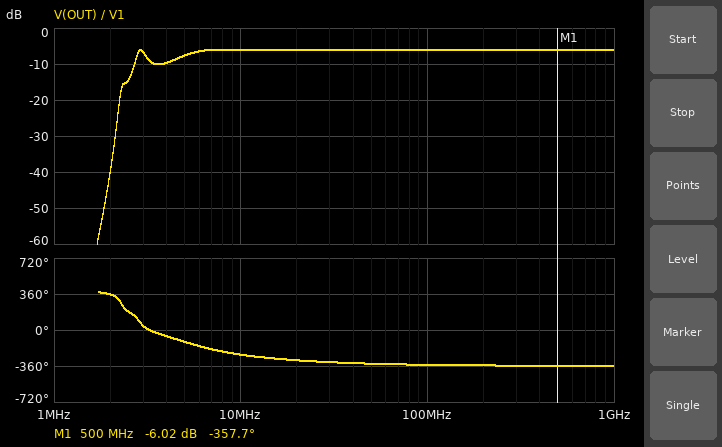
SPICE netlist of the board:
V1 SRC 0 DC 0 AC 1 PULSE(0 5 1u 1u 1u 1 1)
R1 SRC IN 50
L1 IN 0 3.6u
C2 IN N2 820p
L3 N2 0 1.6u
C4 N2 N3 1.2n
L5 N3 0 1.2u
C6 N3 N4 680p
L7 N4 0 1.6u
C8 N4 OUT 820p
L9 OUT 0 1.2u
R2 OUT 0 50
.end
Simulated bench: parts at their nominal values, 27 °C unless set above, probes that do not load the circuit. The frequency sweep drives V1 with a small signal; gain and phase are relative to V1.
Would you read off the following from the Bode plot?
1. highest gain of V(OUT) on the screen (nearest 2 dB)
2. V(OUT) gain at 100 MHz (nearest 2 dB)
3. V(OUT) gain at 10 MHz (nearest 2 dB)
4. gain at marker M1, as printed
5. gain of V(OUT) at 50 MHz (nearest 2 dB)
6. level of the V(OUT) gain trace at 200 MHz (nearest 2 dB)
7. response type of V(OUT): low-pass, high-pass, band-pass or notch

-6 dB
-6 dB
-6 dB
-6.02 dB
-6 dB
-6 dB
high-pass
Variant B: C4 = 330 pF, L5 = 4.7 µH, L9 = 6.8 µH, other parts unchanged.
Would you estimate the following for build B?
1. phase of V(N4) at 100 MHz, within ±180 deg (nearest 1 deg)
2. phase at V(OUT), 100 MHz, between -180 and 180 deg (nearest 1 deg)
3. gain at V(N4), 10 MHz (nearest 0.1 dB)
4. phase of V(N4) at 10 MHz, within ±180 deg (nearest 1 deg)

8 deg
11 deg
-6.4 dB
85 deg
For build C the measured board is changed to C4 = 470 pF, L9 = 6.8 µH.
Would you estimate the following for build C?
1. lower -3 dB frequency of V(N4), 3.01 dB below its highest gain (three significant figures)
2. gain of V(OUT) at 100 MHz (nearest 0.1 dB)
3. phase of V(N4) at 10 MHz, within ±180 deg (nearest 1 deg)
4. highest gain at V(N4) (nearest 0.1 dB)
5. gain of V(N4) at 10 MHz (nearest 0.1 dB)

2.88 MHz
-6.0 dB
92 deg
-5.2 dB
-5.8 dB
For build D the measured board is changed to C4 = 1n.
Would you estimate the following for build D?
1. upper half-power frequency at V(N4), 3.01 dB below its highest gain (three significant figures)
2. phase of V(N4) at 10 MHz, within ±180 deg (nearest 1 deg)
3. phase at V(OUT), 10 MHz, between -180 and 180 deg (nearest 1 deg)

3.11 MHz
88 deg
116 deg
